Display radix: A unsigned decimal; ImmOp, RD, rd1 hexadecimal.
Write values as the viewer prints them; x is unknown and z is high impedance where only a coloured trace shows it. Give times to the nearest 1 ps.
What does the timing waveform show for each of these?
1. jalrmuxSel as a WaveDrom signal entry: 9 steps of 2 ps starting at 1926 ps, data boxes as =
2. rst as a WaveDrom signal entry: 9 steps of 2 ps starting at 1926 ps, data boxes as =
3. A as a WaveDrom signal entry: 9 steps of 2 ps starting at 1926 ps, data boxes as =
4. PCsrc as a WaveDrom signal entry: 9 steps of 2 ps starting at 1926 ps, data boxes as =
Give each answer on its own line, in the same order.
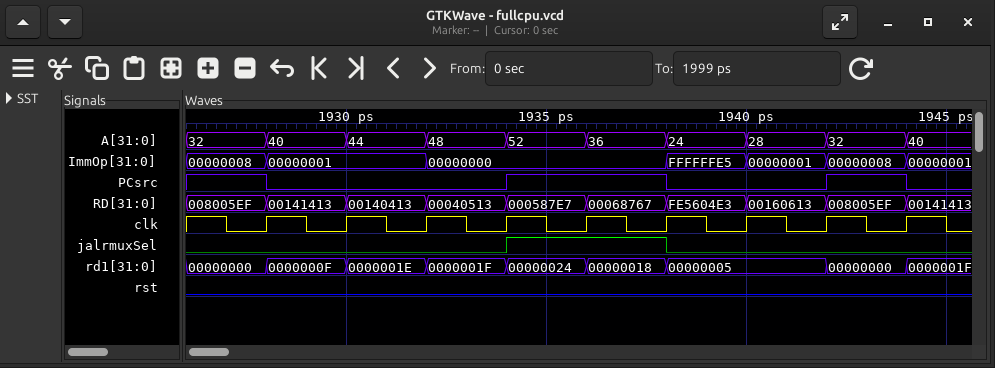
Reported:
{name: 'jalrmuxSel', wave: '0...1.0..'}
{name: 'rst', wave: '0........'}
{name: 'A', wave: '=========', data: '32 40 44 48 52 36 24 28 32'}
{name: 'PCsrc', wave: '10..1.0.1'}
